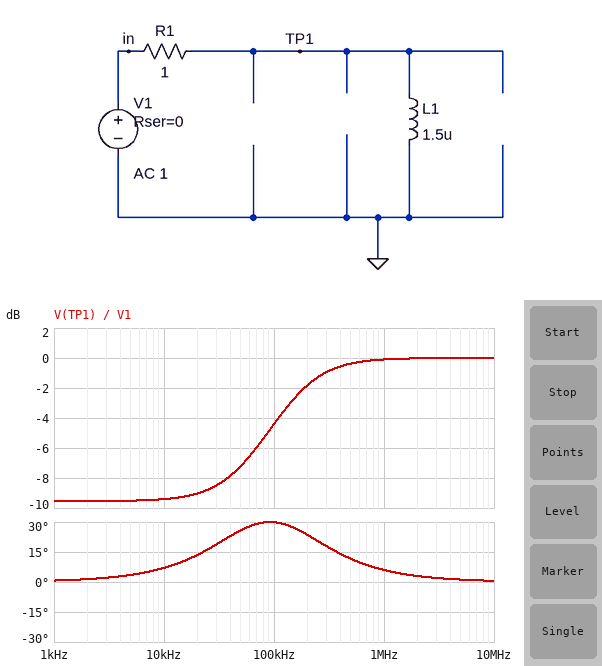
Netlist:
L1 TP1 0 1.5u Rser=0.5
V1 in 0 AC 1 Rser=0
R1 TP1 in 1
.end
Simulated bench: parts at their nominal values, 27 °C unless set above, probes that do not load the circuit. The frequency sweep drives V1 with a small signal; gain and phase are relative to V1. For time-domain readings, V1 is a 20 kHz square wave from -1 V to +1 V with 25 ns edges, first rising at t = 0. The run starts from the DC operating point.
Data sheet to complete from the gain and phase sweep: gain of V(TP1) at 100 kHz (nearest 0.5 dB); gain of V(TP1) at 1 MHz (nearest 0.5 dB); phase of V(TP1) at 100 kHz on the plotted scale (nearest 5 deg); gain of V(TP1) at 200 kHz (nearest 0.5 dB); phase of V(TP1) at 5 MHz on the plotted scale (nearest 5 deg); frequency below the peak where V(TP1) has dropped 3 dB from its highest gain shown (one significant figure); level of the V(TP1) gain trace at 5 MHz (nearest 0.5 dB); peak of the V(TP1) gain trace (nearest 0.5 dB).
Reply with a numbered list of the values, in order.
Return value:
1. -4.5 dB
2. 0 dB
3. 30 deg
4. -2.0 dB
5. 0 deg
6. 100 kHz
7. 0 dB
8. 0 dB
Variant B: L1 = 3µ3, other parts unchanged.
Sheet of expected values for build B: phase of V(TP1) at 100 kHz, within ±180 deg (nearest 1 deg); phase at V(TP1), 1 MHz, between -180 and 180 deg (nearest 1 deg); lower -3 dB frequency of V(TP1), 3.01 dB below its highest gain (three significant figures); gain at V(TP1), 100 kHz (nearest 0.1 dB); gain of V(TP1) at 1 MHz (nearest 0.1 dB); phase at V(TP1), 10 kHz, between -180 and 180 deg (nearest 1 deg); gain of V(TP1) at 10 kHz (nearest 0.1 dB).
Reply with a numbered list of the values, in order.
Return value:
1. 22 deg
2. 3 deg
3. 63.8 kHz
4. -1.6 dB
5. 0 dB
6. 15 deg
7. -8.9 dB
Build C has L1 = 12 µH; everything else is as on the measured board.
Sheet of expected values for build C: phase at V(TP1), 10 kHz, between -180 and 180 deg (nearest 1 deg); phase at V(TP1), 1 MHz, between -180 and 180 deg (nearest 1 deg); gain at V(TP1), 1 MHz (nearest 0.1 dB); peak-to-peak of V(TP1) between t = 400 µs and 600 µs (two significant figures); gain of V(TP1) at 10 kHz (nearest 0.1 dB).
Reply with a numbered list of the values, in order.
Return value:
1. 30 deg
2. 1 deg
3. 0 dB
4. 3.2 V
5. -5.4 dB
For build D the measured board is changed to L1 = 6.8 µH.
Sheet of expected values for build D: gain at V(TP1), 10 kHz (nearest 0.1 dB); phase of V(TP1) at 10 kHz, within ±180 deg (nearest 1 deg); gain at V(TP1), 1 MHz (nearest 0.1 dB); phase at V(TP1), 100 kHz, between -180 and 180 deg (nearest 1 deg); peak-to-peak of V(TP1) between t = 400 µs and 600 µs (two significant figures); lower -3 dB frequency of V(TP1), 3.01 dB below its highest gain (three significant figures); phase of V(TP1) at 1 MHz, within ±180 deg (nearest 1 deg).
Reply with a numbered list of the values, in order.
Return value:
1. -7.5 dB
2. 25 deg
3. 0 dB
4. 13 deg
5. 3.3 V
6. 31.0 kHz
7. 1 deg
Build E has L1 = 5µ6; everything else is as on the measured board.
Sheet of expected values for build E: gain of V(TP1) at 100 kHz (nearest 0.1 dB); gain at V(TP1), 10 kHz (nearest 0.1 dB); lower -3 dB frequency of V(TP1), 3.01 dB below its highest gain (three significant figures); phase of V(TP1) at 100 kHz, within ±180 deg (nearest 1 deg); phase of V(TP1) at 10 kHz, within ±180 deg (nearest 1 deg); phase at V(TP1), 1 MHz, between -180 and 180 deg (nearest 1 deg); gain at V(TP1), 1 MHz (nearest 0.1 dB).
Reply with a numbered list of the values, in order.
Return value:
1. -0.6 dB
2. -8.0 dB
3. 37.6 kHz
4. 15 deg
5. 22 deg
6. 2 deg
7. 0 dB
